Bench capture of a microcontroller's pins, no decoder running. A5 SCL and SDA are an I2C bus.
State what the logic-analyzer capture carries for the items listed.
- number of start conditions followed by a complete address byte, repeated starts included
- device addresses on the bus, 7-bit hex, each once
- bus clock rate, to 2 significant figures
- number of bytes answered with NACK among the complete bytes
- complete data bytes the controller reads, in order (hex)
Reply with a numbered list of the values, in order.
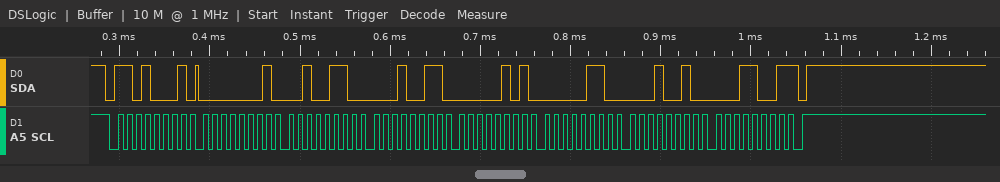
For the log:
1. 1
2. 0x68
3. 100 kHz
4. 1
5. 01 26 13 05 06 12 19
